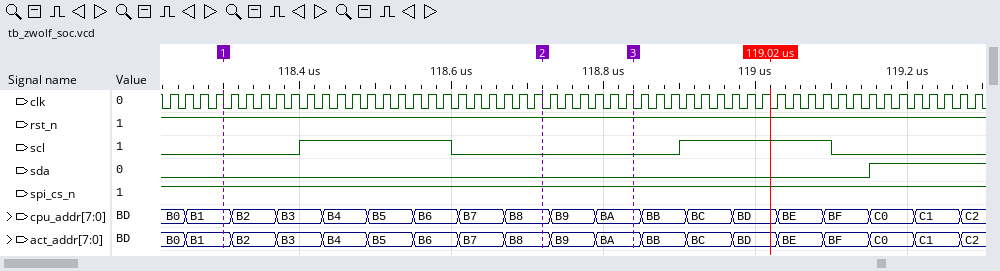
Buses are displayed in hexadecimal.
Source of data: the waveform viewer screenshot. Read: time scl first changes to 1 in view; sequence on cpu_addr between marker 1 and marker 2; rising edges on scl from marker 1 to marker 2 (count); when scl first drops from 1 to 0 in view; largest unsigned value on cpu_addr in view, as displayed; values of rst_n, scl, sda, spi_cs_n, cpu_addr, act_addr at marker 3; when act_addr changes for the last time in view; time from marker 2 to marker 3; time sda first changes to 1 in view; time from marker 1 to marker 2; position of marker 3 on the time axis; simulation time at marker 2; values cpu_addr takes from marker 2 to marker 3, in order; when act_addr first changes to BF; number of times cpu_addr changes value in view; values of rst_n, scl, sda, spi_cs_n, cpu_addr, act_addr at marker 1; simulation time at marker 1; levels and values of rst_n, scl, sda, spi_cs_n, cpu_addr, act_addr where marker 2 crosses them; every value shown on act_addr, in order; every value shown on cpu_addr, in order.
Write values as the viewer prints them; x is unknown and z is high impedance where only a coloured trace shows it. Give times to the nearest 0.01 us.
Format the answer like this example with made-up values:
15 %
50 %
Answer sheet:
118.4 us
B1, B2, B3, B4, B5, B6, B7, B8
1
118.6 us
C2
rst_n=1, scl=0, sda=0, spi_cs_n=1, cpu_addr=BA, act_addr=BA
119.27 us
0.12 us
119.15 us
0.42 us
118.84 us
118.72 us
B8, B9, BA
119.09 us
18
rst_n=1, scl=0, sda=0, spi_cs_n=1, cpu_addr=B1, act_addr=B1
118.3 us
rst_n=1, scl=0, sda=0, spi_cs_n=1, cpu_addr=B8, act_addr=B8
B0, B1, B2, B3, B4, B5, B6, B7, B8, B9, BA, BB, BC, BD, BE, BF, C0, C1, C2
B0, B1, B2, B3, B4, B5, B6, B7, B8, B9, BA, BB, BC, BD, BE, BF, C0, C1, C2
